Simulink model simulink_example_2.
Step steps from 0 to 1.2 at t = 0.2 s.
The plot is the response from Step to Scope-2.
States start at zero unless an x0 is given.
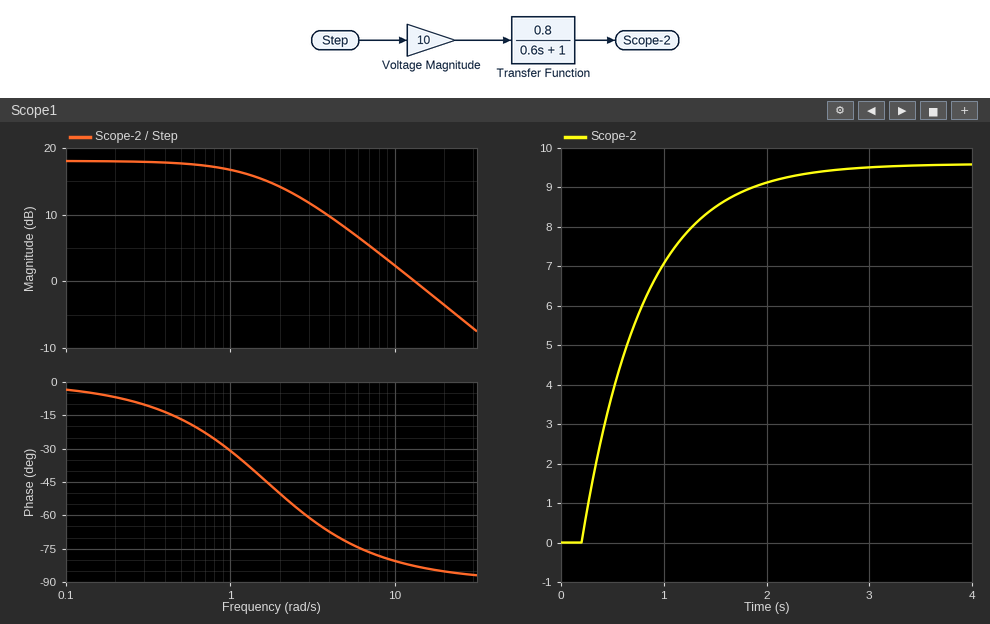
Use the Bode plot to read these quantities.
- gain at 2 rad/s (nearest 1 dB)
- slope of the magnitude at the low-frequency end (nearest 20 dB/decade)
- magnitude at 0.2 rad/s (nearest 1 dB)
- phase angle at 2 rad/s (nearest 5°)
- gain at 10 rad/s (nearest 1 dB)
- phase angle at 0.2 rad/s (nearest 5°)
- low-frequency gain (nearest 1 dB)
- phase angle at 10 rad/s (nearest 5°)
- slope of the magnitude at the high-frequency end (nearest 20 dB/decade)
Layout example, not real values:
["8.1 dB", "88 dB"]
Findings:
["14 dB", "0 dB/decade", "18 dB", "-50°", "2 dB", "-5°", "18 dB", "-80°", "-20 dB/decade"]
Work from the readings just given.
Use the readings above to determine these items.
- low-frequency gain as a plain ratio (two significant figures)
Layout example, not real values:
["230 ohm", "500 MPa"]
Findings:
["7.9"]
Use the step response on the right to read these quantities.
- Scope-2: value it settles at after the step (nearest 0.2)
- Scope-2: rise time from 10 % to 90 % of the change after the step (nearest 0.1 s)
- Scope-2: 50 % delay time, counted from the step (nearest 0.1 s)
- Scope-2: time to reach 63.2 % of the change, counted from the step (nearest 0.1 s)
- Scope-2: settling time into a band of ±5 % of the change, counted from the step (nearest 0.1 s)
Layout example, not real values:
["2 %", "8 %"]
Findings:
["9.6", "1.3 s", "0.4 s", "0.6 s", "1.8 s"]
